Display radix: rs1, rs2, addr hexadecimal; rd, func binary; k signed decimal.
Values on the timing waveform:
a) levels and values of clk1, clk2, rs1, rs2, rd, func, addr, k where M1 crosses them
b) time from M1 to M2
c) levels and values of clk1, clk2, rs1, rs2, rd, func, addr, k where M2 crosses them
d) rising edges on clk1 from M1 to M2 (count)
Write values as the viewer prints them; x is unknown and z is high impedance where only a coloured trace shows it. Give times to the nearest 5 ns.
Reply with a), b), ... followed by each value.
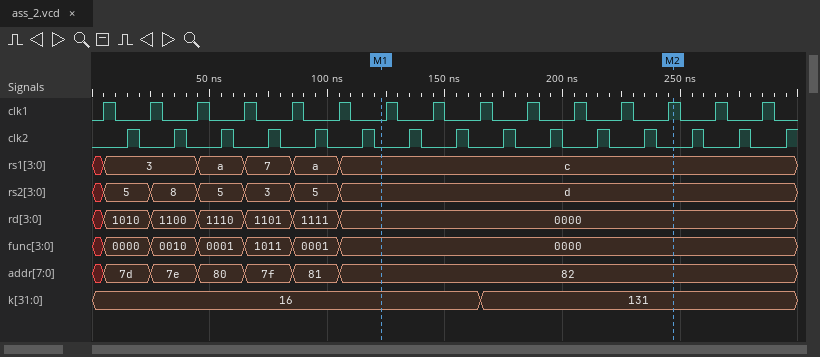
a) clk1=0, clk2=0, rs1=c, rs2=d, rd=0000, func=0000, addr=82, k=16
b) 125 ns
c) clk1=1, clk2=0, rs1=c, rs2=d, rd=0000, func=0000, addr=82, k=131
d) 7
